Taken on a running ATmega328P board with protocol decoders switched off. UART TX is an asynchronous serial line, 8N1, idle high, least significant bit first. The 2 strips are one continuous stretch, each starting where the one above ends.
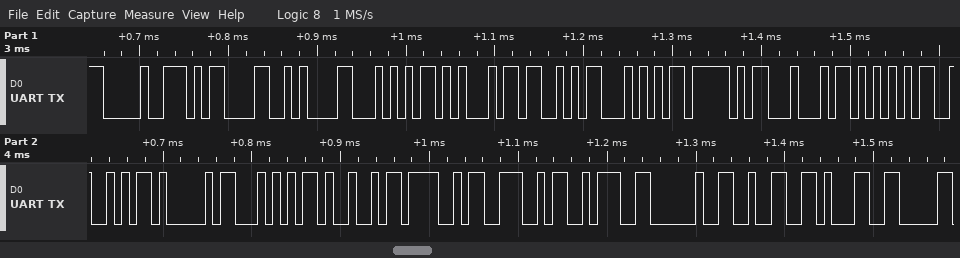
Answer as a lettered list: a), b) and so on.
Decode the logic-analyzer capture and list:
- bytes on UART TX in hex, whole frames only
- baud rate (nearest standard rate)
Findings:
a) 0x90 0x0D 0x0A 0x54 0x45 0x53 0x54 0x5F 0x44 0x55 0x52 0x41 0x54 0x49 0x4F 0x4E 0x3A 0x20 0x32 0x31
b) 115200 baud
